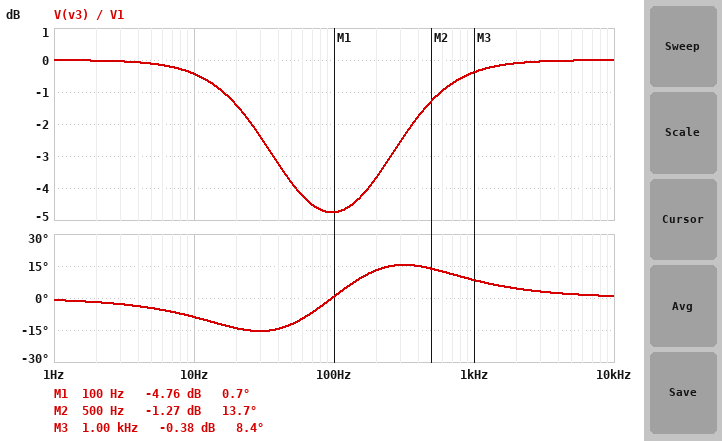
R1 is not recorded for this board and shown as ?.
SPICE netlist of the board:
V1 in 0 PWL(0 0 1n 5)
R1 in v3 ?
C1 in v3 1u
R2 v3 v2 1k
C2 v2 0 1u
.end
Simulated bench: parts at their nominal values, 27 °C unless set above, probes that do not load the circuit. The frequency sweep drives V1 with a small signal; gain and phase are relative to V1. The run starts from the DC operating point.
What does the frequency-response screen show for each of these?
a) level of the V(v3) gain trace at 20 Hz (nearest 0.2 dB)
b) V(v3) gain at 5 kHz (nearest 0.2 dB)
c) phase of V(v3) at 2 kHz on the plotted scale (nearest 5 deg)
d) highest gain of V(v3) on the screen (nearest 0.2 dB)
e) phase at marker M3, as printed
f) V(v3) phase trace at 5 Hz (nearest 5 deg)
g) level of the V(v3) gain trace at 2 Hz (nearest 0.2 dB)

-1.4 dB
0 dB
5 deg
0 dB
8.4 deg
-5 deg
0 dB
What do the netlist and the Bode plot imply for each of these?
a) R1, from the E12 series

2.7 kΩ
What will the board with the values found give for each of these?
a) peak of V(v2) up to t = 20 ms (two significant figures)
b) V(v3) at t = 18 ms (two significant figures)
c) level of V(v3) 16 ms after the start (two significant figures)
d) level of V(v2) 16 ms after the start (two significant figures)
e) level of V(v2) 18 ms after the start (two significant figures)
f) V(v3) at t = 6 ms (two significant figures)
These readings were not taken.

4.9 V
4.9 V
4.8 V
4.8 V
4.9 V
4.1 V
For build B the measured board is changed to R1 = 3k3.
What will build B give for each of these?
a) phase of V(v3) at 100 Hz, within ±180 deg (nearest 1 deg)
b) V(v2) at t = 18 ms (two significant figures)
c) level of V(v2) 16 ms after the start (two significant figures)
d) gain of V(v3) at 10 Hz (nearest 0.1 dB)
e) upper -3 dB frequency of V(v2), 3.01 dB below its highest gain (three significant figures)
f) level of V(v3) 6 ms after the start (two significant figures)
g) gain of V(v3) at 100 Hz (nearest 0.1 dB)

3 deg
4.8 V
4.7 V
-0.6 dB
29.2 Hz
3.9 V
-4.9 dB
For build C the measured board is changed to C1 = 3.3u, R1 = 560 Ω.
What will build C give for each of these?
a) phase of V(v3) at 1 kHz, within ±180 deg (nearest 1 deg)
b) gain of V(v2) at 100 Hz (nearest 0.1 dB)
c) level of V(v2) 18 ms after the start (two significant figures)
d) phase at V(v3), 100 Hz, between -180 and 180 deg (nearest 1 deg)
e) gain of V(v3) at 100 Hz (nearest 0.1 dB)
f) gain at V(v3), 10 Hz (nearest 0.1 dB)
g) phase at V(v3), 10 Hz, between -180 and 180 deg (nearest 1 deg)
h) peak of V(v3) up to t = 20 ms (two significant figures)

3 deg
-3.0 dB
5.0 V
-1 deg
-1.5 dB
-0.1 dB
-2 deg
5.0 V
